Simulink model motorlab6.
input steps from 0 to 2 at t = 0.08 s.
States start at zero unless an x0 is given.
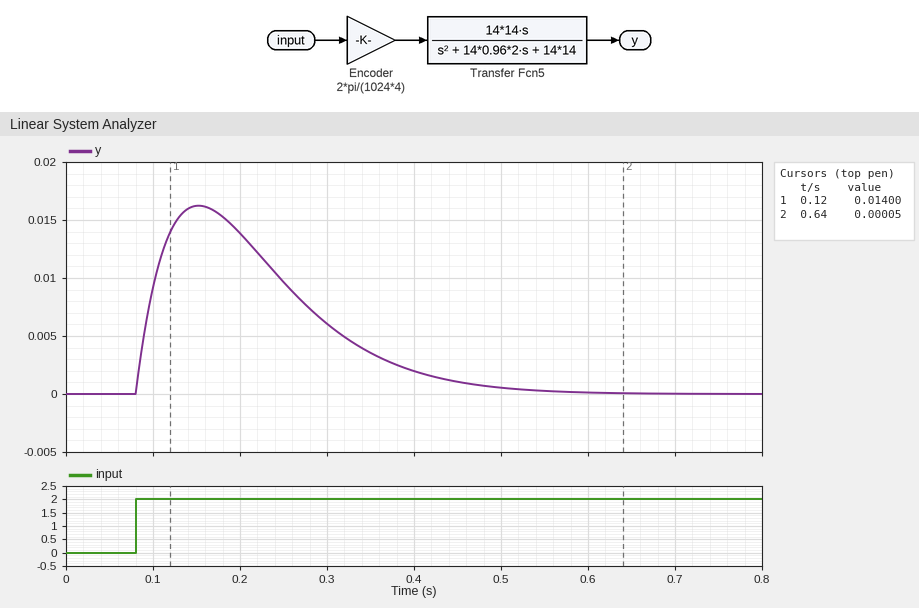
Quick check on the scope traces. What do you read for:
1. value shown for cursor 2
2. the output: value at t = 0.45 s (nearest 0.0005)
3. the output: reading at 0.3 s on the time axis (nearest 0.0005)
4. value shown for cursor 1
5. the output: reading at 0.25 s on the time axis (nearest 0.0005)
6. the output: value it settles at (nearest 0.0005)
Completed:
0.00005
0.0010
0.0060
0.01400
0.0095
0.0000
